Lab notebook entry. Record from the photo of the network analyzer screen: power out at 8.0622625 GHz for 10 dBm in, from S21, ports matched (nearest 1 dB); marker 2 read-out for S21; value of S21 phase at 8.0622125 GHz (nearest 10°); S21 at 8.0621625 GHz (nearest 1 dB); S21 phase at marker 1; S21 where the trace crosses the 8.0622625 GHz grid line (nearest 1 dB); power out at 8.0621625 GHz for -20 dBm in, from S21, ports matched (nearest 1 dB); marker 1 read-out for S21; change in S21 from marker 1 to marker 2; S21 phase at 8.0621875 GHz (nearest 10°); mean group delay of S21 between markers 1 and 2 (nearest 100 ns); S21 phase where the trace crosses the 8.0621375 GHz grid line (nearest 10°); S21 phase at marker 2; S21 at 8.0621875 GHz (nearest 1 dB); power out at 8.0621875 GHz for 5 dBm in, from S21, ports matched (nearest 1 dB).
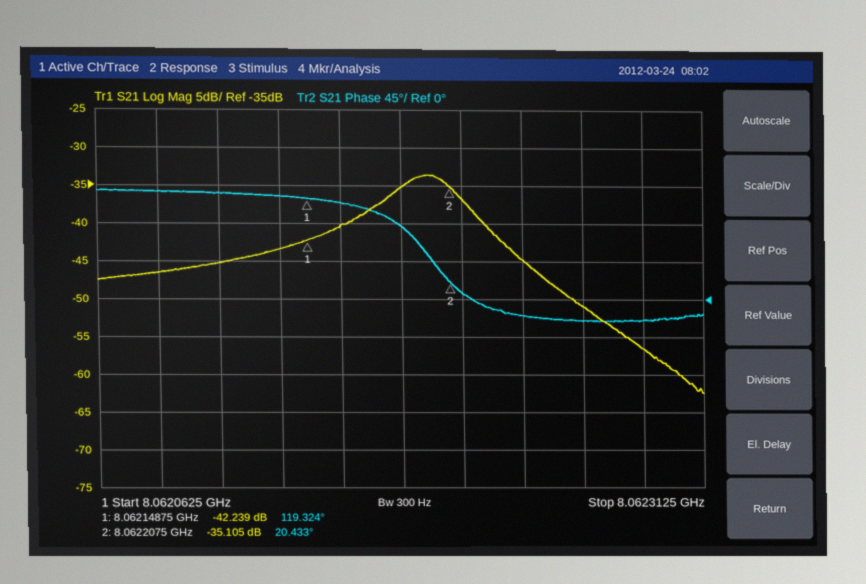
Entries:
-41 dBm
-35.105 dB
10°
-40 dB
119.324°
-51 dB
-60 dBm
-42.239 dB
7.134 dB
90°
4.7 µs
120°
20.433°
-35 dB
-30 dBm
